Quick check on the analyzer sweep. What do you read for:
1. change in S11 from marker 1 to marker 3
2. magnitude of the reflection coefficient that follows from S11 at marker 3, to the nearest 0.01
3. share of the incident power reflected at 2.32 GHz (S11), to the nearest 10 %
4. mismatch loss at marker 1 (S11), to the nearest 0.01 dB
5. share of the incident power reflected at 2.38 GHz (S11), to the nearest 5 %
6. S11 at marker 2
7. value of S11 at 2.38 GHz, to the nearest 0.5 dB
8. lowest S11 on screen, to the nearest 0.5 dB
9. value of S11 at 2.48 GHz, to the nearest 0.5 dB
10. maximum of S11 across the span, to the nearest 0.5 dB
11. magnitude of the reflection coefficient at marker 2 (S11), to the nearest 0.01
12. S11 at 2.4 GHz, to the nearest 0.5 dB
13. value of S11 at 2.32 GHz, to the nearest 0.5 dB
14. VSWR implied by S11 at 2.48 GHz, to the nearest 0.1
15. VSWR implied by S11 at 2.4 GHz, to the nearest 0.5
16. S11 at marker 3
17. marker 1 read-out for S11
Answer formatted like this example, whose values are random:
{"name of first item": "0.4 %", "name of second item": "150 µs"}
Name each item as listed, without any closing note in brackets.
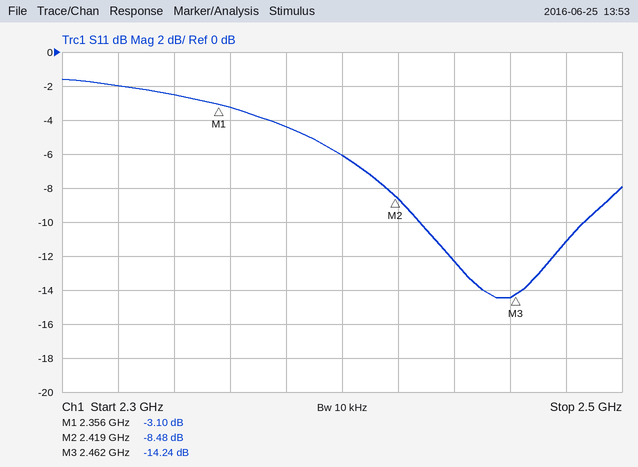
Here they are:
{"change in S11 from marker 1 to marker 3": "-11.14 dB", "magnitude of the reflection coefficient that follows from S11 at marker 3, to the nearest 0.01": "0.19", "share of the incident power reflected at 2.32 GHz (S11), to the nearest 10 %": "60 %", "mismatch loss at marker 1 (S11), to the nearest 0.01 dB": "2.92 dB", "share of the incident power reflected at 2.38 GHz (S11), to the nearest 5 %": "35 %", "S11 at marker 2": "-8.48 dB", "value of S11 at 2.38 GHz, to the nearest 0.5 dB": "-4.5 dB", "lowest S11 on screen, to the nearest 0.5 dB": "-14.5 dB", "value of S11 at 2.48 GHz, to the nearest 0.5 dB": "-11.0 dB", "maximum of S11 across the span, to the nearest 0.5 dB": "-1.5 dB", "magnitude of the reflection coefficient at marker 2 (S11), to the nearest 0.01": "0.38", "S11 at 2.4 GHz, to the nearest 0.5 dB": "-6.0 dB", "value of S11 at 2.32 GHz, to the nearest 0.5 dB": "-2.0 dB", "VSWR implied by S11 at 2.48 GHz, to the nearest 0.1": "1.8", "VSWR implied by S11 at 2.4 GHz, to the nearest 0.5": "3.0", "S11 at marker 3": "-14.24 dB", "marker 1 read-out for S11": "-3.10 dB"}
